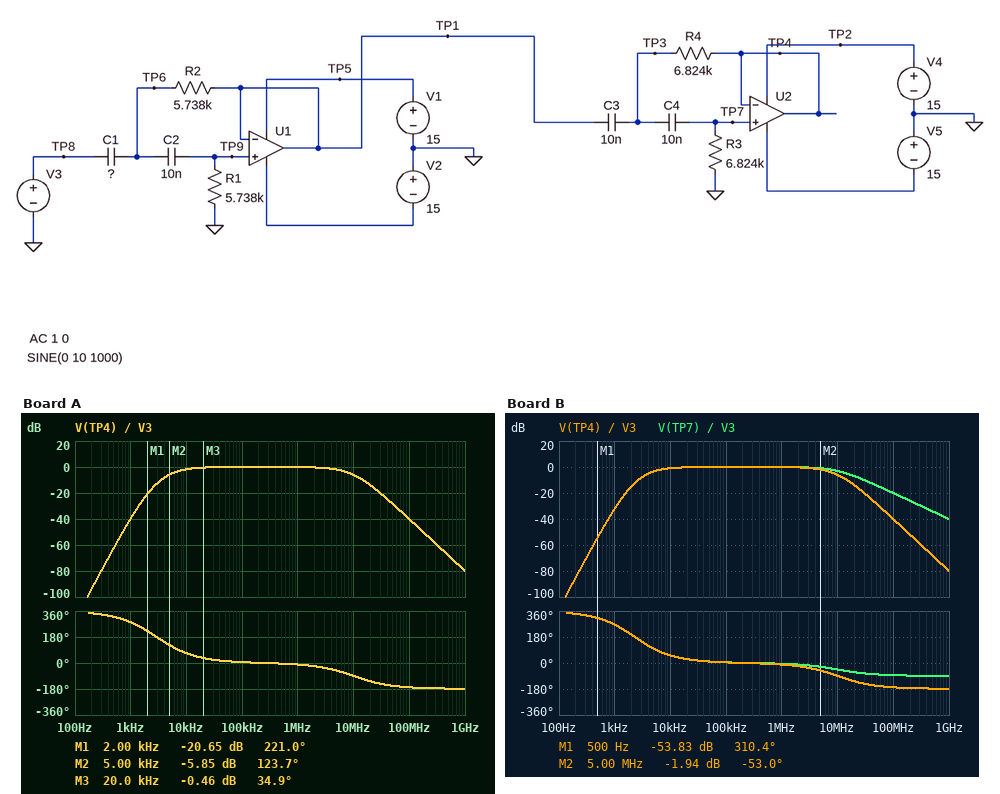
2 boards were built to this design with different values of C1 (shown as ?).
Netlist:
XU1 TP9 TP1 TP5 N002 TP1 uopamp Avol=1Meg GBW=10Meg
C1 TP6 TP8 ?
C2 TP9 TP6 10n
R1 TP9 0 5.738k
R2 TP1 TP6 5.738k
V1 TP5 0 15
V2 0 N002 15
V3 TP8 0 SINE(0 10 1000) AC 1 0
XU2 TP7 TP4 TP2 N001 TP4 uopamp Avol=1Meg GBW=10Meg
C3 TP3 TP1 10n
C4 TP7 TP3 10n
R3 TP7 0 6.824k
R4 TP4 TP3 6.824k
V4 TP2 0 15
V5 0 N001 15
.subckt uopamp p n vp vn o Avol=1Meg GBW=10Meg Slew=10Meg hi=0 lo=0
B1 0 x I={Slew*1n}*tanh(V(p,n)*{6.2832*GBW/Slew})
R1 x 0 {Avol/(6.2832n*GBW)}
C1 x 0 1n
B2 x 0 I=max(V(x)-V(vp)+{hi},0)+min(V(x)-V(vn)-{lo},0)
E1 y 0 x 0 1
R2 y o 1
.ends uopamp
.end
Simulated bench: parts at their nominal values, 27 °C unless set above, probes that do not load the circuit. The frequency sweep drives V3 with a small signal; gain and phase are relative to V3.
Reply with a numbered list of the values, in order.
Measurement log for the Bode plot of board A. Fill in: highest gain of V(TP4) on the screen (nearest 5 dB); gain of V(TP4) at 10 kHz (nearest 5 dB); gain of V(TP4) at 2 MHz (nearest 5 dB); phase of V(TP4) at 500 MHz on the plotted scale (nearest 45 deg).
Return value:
1. 0 dB
2. 0 dB
3. 0 dB
4. -180 deg
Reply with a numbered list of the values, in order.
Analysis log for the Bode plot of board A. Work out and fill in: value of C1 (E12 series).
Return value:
1. 5.6 nF
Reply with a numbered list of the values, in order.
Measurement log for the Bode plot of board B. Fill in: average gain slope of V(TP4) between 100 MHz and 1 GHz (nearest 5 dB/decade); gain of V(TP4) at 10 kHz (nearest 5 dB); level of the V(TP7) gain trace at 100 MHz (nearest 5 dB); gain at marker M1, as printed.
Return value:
1. -40 dB/decade
2. 0 dB
3. -20 dB
4. -53.83 dB
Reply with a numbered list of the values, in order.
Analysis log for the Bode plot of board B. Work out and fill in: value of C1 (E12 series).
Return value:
1. 15 nF
